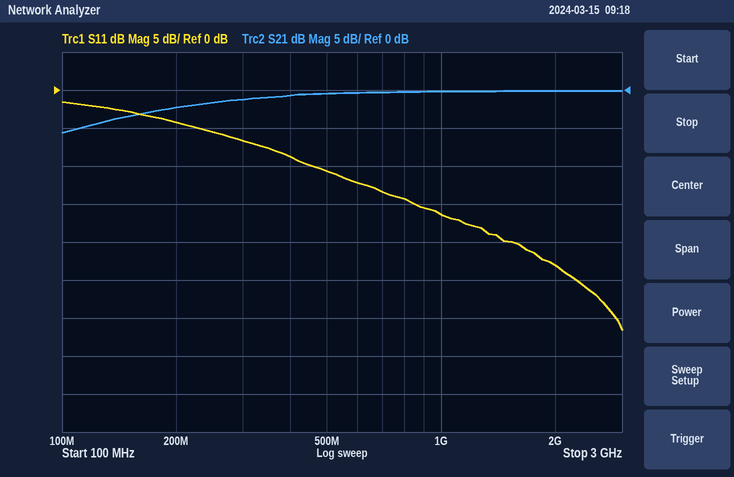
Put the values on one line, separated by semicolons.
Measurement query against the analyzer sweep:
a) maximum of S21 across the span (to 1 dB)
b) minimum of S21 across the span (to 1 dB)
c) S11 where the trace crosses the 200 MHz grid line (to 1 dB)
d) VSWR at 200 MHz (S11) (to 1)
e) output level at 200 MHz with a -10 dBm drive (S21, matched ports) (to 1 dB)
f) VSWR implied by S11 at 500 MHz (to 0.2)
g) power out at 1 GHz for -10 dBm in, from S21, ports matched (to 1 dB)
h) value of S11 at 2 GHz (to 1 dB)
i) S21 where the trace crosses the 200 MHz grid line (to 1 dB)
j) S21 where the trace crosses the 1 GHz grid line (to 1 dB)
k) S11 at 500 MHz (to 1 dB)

0 dB; -6 dB; -4 dB; 4; -12 dBm; 1.8; -10 dBm; -23 dB; -2 dB; 0 dB; -11 dB
